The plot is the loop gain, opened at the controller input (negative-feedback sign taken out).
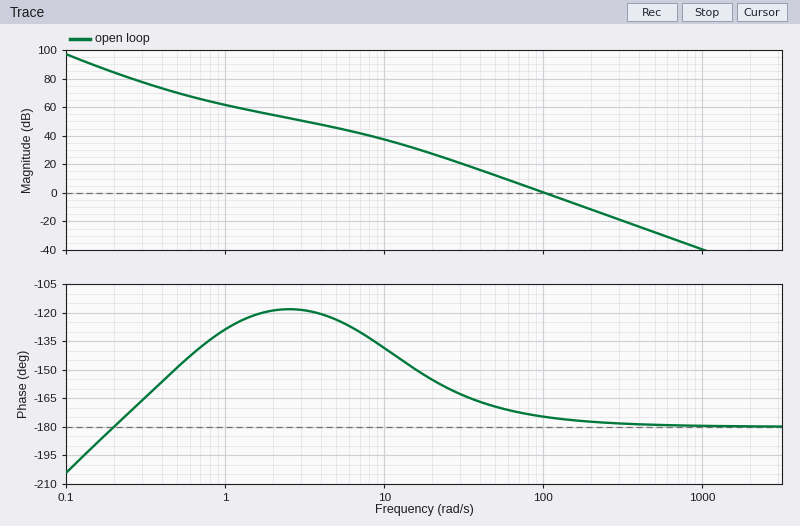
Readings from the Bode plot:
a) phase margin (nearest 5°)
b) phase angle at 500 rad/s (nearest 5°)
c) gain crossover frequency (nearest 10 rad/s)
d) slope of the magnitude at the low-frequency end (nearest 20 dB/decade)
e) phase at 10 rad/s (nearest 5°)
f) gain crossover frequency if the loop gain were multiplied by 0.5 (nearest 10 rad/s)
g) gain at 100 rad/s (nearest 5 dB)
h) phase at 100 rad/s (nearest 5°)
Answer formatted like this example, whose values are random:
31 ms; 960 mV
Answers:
5°; -180°; 100 rad/s; -40 dB/decade; -140°; 70 rad/s; 0 dB; -175°
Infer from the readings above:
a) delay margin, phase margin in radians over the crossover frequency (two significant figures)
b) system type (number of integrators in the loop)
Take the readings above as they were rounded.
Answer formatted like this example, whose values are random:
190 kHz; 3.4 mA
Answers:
0.00087 s; 2
